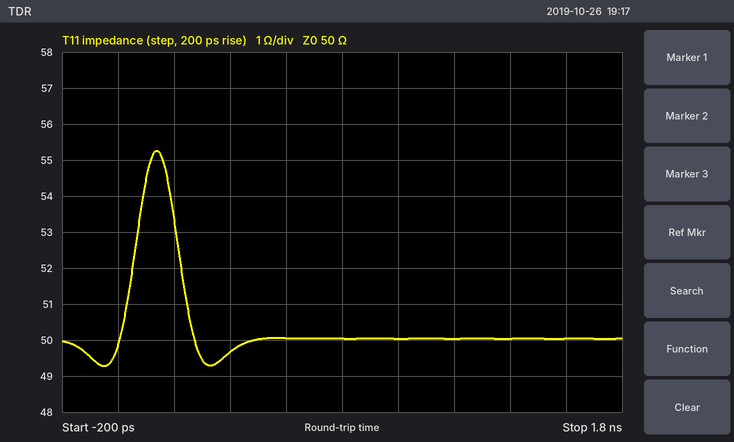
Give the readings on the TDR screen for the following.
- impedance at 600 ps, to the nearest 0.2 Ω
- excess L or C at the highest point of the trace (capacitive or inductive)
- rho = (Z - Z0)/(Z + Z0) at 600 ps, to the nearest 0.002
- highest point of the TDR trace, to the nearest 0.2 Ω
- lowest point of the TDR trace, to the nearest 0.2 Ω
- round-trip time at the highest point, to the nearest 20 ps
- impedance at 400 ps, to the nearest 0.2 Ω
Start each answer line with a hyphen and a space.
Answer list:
- 50.0 Ω
- inductive
- 0.000
- 55.2 Ω
- 49.2 Ω
- 140 ps
- 49.6 Ω
